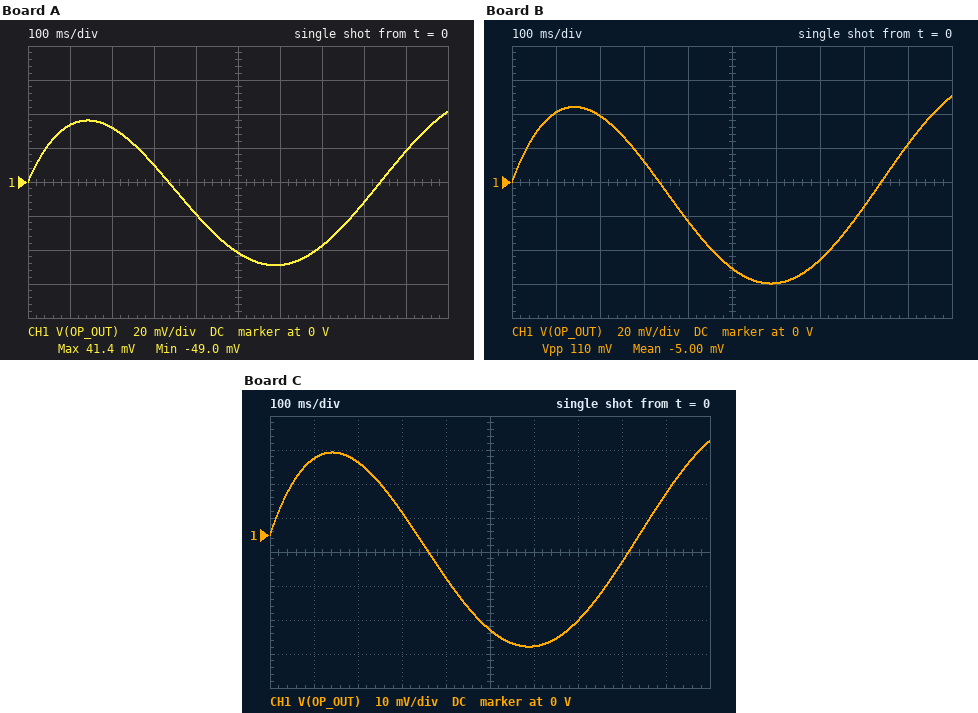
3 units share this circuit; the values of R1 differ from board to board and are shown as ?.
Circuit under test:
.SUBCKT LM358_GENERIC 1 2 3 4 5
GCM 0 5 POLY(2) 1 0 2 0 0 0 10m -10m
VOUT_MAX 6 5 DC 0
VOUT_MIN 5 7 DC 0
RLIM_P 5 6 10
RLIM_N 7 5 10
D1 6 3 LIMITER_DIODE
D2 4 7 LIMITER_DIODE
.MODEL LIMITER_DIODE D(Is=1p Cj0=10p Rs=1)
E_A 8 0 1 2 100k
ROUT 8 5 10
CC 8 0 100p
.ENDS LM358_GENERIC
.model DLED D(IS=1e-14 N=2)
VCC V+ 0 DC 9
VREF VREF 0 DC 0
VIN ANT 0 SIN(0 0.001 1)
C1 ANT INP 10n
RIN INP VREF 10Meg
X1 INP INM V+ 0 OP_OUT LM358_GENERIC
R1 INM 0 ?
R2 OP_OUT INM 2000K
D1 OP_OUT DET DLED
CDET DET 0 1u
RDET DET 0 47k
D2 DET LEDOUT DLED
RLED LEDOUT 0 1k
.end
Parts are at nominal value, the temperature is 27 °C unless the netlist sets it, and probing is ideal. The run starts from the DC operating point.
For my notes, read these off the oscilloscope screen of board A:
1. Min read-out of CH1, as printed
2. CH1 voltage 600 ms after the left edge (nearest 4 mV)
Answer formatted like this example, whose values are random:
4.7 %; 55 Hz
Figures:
-49.0 mV; -48 mV
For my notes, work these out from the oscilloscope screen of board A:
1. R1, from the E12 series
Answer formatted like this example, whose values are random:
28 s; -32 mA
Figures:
22 kΩ
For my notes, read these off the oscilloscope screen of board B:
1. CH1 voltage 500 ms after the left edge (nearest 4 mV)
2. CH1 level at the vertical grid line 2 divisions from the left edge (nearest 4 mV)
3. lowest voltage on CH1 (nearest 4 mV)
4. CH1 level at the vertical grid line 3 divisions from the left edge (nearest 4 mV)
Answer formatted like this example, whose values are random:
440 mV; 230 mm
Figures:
-52 mV; 40 mV; -60 mV; 12 mV
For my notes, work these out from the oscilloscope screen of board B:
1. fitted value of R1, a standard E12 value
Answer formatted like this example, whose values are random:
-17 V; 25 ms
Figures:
18 kΩ
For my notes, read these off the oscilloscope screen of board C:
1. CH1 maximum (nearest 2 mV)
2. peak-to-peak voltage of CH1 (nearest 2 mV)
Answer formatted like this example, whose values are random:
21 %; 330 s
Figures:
28 mV; 60 mV
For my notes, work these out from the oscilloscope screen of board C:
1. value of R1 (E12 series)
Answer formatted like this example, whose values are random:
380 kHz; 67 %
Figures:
33 kΩ
